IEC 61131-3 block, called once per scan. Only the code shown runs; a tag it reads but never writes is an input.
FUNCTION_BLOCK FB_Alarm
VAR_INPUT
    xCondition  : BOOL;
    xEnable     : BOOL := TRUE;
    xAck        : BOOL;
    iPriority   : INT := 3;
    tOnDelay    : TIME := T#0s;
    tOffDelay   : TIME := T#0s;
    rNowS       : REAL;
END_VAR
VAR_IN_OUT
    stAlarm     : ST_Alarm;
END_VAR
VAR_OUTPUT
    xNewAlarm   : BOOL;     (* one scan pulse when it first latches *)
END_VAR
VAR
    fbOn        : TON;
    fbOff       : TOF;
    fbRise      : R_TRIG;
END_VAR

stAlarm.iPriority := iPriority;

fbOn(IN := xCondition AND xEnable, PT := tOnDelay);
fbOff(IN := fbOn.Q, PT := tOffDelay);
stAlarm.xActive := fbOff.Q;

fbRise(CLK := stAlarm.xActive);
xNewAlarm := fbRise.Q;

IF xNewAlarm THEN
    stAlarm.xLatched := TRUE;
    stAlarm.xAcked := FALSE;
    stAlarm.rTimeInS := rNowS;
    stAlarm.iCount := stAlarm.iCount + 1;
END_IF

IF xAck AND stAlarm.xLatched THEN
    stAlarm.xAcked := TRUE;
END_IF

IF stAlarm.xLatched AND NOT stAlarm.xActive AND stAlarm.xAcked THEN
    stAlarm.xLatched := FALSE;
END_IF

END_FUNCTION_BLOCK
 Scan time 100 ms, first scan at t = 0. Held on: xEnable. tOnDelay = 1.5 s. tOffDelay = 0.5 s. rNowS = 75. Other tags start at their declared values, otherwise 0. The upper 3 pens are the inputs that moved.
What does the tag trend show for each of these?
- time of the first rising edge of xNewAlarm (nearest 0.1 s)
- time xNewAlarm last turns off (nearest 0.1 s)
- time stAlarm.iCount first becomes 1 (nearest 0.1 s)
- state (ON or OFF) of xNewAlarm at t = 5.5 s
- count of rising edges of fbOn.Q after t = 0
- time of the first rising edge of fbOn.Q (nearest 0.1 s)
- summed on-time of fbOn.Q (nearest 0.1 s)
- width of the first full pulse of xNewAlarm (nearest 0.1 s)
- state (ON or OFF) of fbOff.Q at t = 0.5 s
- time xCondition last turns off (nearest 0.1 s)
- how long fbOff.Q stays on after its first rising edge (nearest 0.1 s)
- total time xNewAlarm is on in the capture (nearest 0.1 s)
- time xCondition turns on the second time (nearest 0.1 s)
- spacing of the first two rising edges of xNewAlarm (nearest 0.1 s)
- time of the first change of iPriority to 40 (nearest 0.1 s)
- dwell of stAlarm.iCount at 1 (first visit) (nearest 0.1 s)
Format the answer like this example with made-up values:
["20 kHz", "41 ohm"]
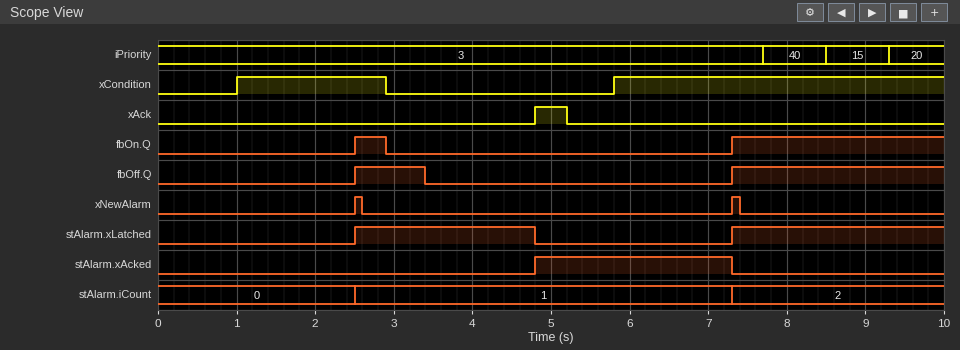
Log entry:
["2.5 s", "7.4 s", "2.5 s", "OFF", "2", "2.5 s", "3.1 s", "0.1 s", "OFF", "2.9 s", "0.9 s", "0.2 s", "5.8 s", "4.8 s", "7.7 s", "4.8 s"]
